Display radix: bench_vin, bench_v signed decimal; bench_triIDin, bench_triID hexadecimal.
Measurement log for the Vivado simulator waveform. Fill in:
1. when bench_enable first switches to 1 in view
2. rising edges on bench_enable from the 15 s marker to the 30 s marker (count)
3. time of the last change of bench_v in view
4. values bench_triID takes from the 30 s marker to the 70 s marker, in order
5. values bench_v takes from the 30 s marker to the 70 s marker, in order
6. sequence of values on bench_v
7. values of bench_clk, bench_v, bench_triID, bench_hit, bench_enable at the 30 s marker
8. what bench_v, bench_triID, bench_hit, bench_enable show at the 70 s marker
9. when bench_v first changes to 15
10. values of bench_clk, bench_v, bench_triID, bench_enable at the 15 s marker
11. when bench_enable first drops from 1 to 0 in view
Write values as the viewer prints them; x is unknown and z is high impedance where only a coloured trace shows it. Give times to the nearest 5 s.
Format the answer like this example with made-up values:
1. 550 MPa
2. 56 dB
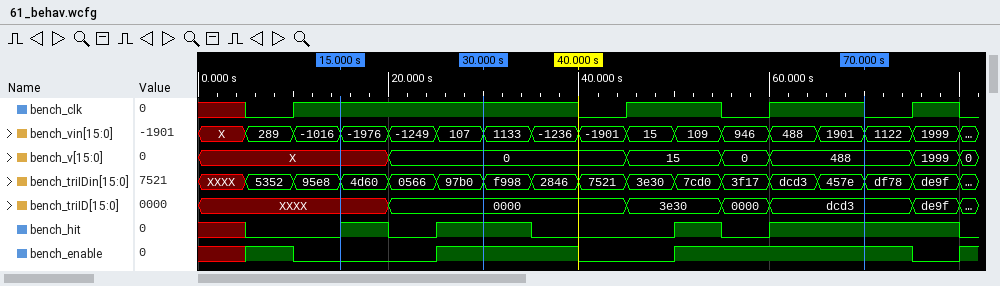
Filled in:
1. 5 s
2. 1
3. 80 s
4. 0000, 3e30, 0000, dcd3
5. 0, 15, 0, 488
6. X, 0, 15, 0, 488, 1999, 0
7. bench_clk=1, bench_v=0, bench_triID=0000, bench_hit=1, bench_enable=1
8. bench_v=488, bench_triID=dcd3, bench_hit=1, bench_enable=1
9. 45 s
10. bench_clk=1, bench_v=X, bench_triID=XXXX, bench_enable=0
11. 10 s
